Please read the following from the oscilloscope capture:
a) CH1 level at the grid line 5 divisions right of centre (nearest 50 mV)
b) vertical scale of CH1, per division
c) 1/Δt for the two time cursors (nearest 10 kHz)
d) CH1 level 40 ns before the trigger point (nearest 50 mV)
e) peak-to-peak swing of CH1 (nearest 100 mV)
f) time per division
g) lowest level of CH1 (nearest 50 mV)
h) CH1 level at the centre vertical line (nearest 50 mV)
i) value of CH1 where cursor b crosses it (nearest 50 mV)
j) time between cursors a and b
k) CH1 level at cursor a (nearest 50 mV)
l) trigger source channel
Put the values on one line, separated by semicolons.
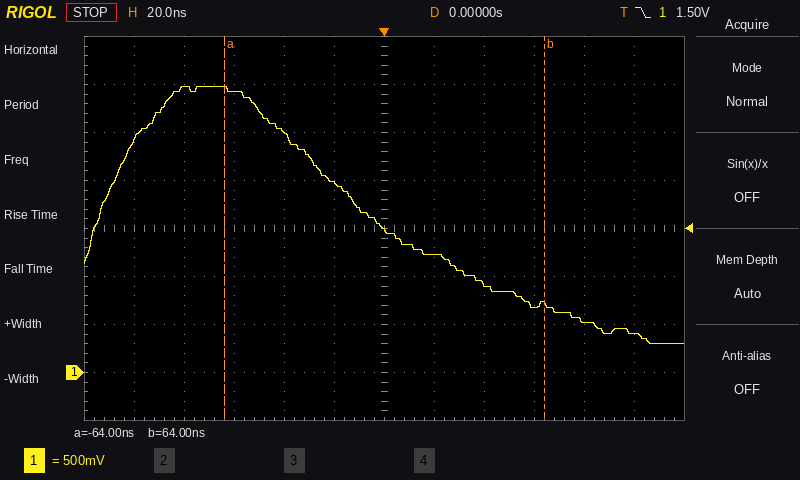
400 mV; 500 mV; 7.81 MHz; 2.50 V; 2.70 V; 20 ns; 300 mV; 1.50 V; 700 mV; 128 ns; 2.95 V; CH1
